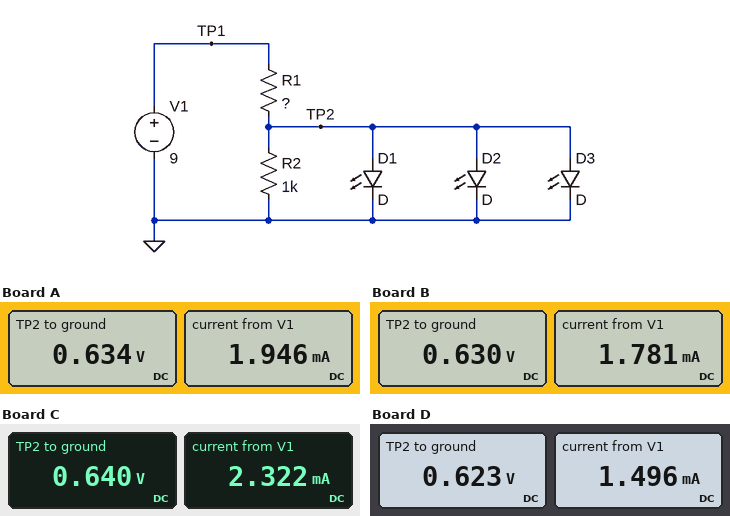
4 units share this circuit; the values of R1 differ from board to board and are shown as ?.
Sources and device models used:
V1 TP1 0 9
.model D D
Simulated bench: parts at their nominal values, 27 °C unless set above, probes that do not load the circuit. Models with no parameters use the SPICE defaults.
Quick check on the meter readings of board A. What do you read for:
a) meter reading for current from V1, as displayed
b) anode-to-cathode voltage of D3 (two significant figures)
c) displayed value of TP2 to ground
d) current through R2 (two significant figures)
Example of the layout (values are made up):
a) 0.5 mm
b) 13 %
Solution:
a) 1.946 mA
b) 630 mV
c) 0.634 V
d) 630 µA
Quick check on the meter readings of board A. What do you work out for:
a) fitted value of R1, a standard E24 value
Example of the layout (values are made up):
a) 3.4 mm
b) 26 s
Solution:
a) 4.3 kΩ
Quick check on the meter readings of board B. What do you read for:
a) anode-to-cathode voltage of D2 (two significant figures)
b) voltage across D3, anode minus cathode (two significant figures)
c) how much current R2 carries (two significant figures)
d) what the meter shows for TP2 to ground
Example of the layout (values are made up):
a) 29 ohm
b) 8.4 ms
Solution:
a) 630 mV
b) 630 mV
c) 630 µA
d) 0.630 V
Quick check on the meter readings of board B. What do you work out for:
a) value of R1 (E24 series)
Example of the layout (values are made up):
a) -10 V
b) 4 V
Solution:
a) 4.7 kΩ
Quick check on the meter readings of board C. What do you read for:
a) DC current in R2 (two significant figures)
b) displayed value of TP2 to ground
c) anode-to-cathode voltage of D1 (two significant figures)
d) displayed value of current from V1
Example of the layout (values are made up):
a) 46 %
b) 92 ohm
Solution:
a) 640 µA
b) 0.640 V
c) 640 mV
d) 2.322 mA
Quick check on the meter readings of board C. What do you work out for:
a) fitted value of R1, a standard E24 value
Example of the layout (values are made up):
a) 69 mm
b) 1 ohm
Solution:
a) 3.6 kΩ
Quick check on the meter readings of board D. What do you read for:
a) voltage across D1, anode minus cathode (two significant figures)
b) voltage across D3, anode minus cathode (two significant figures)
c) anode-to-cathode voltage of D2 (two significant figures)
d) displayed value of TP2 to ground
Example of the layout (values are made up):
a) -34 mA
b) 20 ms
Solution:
a) 620 mV
b) 620 mV
c) 620 mV
d) 0.623 V
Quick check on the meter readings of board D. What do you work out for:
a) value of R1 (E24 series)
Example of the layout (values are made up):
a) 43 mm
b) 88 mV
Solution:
a) 5.6 kΩ
